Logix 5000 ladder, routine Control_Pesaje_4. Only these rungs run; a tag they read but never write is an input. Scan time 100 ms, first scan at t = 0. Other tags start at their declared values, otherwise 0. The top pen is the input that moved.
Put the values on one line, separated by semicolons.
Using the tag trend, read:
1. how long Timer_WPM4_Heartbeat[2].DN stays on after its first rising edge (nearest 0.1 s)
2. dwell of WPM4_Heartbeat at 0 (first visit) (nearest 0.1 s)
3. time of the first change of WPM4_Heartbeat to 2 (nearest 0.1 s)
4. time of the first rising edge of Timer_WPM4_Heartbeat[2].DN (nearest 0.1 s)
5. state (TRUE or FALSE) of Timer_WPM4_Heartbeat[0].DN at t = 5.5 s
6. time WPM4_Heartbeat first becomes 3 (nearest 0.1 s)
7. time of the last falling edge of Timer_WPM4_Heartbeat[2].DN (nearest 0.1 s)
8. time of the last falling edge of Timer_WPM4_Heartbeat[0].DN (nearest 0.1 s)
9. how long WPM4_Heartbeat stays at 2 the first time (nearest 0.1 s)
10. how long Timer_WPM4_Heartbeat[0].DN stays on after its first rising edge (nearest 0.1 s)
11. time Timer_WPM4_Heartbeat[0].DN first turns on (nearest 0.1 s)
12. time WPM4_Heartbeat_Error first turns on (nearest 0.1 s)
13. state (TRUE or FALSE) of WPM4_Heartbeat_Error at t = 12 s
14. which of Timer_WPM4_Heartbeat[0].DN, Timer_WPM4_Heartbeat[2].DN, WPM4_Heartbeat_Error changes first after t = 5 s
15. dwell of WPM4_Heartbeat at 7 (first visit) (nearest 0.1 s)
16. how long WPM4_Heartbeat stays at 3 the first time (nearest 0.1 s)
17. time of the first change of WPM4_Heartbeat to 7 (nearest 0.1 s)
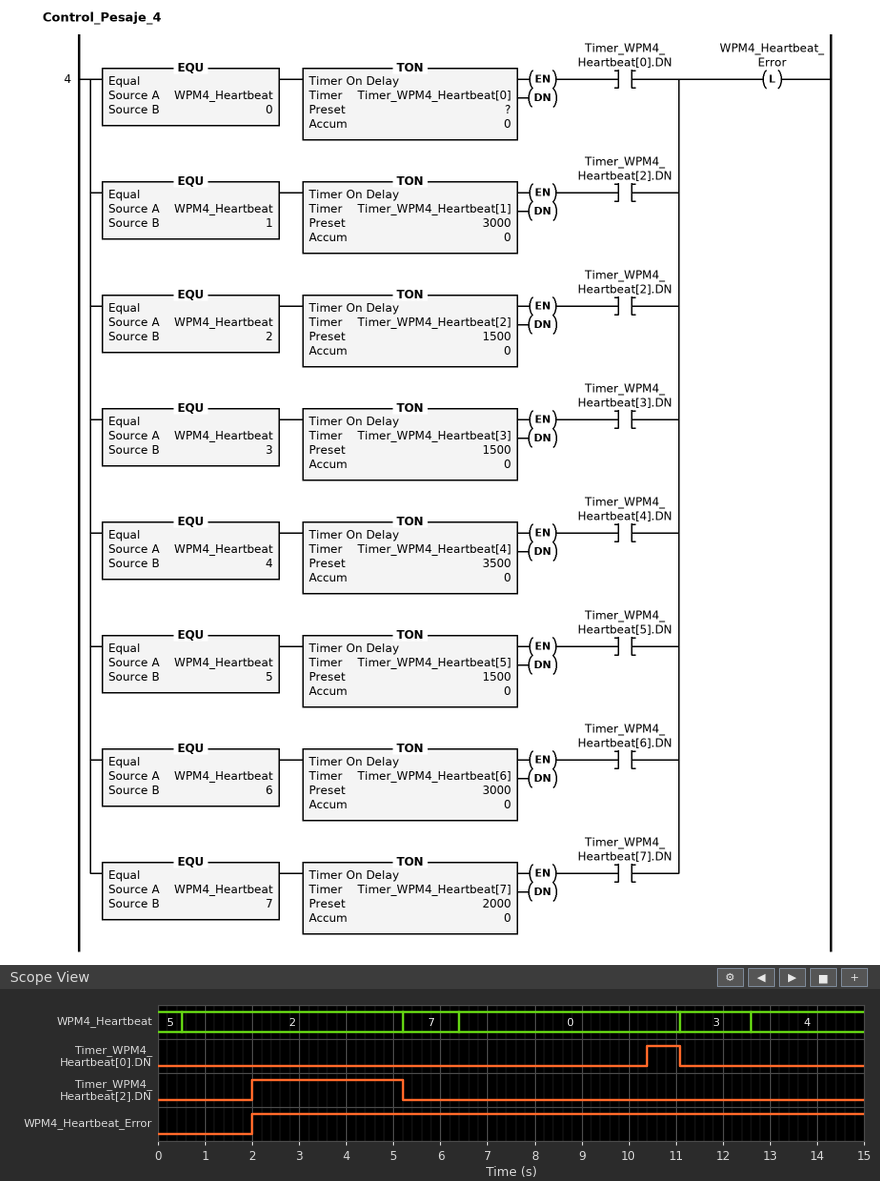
3.2 s; 4.7 s; 0.5 s; 2.0 s; FALSE; 11.1 s; 5.2 s; 11.1 s; 4.7 s; 0.7 s; 10.4 s; 2.0 s; TRUE; Timer_WPM4_Heartbeat[2].DN; 1.2 s; 1.5 s; 5.2 s
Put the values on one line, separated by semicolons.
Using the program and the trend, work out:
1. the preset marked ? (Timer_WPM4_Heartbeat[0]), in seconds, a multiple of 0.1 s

4.0 s
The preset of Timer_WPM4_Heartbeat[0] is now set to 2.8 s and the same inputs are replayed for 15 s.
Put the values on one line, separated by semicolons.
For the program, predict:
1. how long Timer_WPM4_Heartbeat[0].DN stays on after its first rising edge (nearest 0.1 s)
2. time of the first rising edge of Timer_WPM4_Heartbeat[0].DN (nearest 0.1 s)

1.9 s; 9.2 s
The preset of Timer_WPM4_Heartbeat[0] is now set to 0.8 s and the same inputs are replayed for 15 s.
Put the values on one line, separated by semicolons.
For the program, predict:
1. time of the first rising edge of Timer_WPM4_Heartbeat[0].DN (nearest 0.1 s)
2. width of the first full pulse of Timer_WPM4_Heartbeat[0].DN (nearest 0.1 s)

7.2 s; 3.9 s
